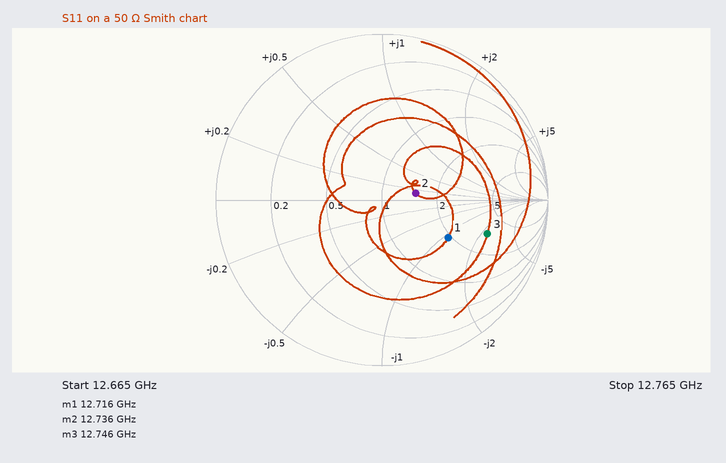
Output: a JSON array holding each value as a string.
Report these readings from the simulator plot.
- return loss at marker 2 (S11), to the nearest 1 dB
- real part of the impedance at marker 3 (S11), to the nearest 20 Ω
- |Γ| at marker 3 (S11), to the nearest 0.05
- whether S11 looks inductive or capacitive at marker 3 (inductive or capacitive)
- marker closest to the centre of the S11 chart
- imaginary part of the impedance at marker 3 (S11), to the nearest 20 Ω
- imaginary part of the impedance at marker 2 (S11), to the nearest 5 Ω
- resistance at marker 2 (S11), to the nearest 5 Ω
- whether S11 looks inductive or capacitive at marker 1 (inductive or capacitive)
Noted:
["14 dB", "160 Ω", "0.65", "capacitive", "marker 2", "-120 Ω", "+5 Ω", "75 Ω", "capacitive"]
